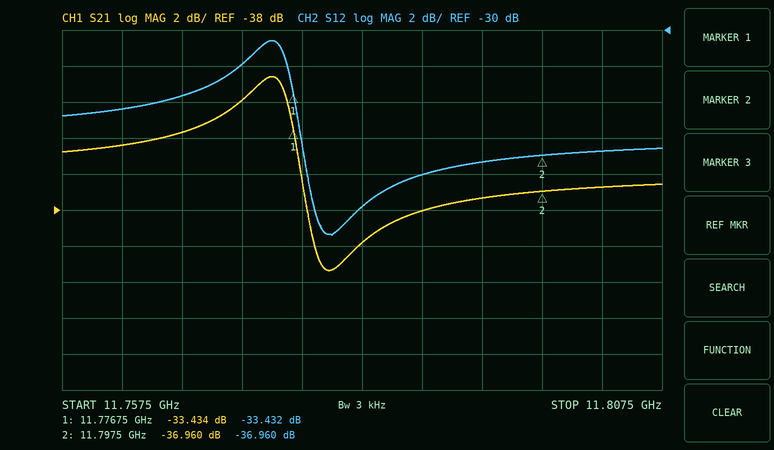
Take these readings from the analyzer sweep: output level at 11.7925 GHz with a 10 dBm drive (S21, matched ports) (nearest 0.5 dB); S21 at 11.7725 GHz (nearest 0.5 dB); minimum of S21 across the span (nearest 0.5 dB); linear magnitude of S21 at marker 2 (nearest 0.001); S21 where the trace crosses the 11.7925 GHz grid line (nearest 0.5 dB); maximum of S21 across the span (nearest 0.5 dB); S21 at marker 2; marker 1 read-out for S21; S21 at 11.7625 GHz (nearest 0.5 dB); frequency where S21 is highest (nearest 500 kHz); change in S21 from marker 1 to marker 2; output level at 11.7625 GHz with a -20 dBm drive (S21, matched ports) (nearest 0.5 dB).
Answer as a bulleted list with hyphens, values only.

- -27.5 dBm
- -32.0 dB
- -41.5 dB
- 0.014
- -37.5 dB
- -30.5 dB
- -36.960 dB
- -33.434 dB
- -34.5 dB
- 11.7750 GHz
- -3.526 dB
- -54.5 dBm
